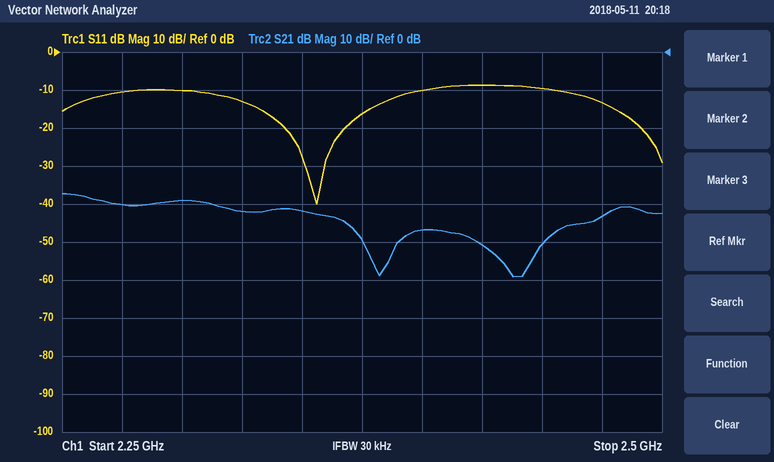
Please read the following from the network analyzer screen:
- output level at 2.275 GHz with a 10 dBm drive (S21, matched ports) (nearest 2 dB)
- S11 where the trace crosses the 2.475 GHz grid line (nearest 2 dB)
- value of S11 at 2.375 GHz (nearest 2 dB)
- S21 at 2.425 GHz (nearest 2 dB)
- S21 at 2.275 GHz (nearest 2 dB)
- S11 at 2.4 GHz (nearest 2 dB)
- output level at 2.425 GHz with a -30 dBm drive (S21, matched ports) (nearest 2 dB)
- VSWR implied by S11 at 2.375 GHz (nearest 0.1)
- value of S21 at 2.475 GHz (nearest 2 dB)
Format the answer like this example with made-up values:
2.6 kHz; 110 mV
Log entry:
-30 dBm; -14 dB; -16 dB; -50 dB; -40 dB; -10 dB; -80 dBm; 1.4; -44 dB
